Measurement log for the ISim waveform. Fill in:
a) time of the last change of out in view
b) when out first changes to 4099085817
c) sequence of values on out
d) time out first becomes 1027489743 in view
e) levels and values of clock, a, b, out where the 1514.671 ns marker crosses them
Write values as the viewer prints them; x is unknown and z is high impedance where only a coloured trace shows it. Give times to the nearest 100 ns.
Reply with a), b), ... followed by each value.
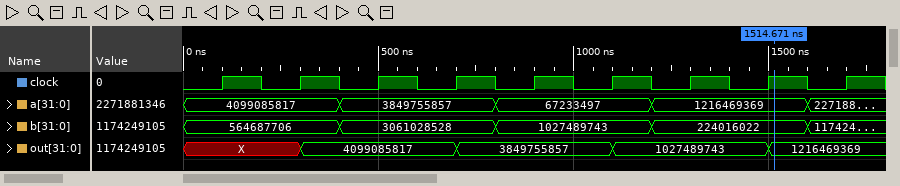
a) 1500 ns
b) 300 ns
c) X, 4099085817, 3849755857, 1027489743, 1216469369
d) 1100 ns
e) clock=1, a=1216469369, b=224016022, out=1216469369
